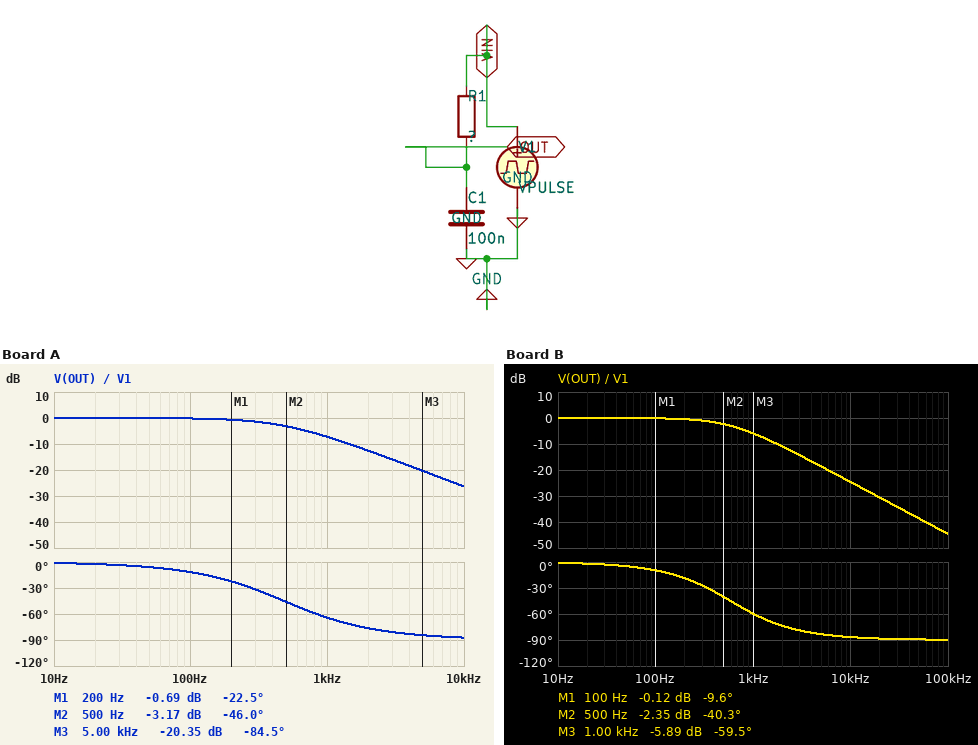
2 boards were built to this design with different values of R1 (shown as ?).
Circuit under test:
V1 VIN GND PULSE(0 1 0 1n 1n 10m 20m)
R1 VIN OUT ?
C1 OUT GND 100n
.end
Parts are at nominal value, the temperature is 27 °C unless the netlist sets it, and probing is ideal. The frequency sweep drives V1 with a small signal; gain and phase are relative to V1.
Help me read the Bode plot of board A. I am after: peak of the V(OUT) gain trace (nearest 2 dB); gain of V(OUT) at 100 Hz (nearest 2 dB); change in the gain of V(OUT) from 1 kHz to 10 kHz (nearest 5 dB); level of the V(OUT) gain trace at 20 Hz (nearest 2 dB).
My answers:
0 dB
0 dB
-20 dB
0 dB
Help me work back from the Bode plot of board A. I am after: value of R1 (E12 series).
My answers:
3.3 kΩ
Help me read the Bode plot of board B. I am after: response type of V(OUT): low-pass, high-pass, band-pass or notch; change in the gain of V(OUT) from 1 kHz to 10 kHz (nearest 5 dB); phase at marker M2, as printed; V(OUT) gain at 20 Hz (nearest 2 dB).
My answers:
low-pass
-20 dB
-40.3 deg
0 dB
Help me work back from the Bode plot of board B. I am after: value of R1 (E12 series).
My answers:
2.7 kΩ
